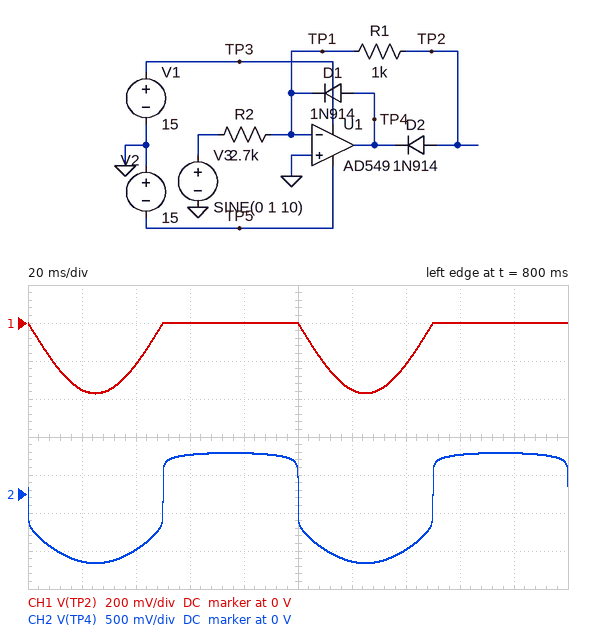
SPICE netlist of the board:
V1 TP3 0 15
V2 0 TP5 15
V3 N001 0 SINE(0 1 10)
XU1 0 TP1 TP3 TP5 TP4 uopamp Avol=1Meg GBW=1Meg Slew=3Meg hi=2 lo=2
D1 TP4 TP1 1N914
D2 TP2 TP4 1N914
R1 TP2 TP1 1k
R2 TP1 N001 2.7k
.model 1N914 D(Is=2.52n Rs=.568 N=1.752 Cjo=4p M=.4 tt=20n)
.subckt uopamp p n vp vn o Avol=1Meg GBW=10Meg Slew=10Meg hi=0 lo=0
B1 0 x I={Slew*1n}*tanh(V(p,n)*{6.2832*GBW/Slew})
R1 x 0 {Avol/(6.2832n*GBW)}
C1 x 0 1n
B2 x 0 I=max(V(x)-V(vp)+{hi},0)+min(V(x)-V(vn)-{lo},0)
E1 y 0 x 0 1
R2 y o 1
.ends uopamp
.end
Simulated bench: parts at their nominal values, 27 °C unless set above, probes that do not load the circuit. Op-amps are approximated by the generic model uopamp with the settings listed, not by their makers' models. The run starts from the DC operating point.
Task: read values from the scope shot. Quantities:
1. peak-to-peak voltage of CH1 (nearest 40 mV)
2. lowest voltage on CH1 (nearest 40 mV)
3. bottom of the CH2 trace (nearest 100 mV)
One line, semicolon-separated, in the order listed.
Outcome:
360 mV; -360 mV; -900 mV
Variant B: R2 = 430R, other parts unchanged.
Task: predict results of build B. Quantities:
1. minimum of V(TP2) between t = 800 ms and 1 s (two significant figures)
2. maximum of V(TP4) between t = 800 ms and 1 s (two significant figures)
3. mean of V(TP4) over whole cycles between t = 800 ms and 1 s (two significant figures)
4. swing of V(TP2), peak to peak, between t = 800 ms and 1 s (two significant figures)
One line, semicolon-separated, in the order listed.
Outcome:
-2.3 V; 620 mV; -740 mV; 2.3 V
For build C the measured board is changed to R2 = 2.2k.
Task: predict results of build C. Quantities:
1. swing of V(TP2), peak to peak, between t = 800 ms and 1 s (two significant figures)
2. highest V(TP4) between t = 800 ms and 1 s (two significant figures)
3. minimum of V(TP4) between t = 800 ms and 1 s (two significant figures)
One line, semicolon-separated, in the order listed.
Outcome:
460 mV; 550 mV; -1.0 V
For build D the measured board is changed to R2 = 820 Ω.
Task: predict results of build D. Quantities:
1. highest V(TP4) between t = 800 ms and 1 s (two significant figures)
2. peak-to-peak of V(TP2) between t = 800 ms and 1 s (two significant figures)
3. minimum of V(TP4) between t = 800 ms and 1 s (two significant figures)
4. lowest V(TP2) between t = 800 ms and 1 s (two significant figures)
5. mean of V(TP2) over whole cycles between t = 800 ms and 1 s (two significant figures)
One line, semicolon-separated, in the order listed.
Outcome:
590 mV; 1.2 V; -1.8 V; -1.2 V; -390 mV
